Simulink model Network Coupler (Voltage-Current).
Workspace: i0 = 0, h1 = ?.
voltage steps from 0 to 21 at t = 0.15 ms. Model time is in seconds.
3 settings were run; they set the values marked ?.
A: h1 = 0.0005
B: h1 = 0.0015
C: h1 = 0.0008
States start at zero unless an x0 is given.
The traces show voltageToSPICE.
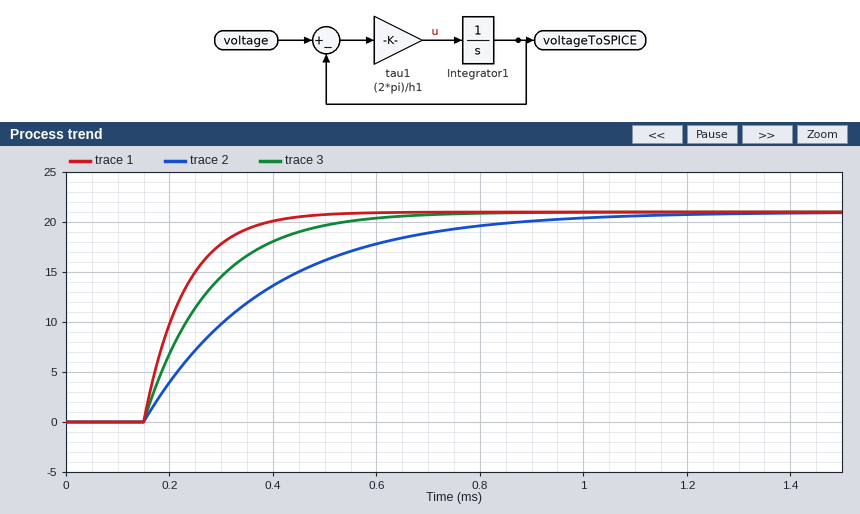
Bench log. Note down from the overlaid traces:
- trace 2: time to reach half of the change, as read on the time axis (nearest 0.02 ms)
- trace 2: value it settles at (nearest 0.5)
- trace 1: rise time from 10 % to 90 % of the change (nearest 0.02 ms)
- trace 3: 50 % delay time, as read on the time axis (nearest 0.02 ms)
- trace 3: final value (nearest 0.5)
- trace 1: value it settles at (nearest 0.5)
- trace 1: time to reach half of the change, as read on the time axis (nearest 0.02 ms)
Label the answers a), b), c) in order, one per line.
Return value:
a) 0.32 ms
b) 21.0
c) 0.18 ms
d) 0.24 ms
e) 21.0
f) 21.0
g) 0.20 ms
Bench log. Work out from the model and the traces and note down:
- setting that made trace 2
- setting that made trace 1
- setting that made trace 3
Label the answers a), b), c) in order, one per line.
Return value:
a) B
b) A
c) C
